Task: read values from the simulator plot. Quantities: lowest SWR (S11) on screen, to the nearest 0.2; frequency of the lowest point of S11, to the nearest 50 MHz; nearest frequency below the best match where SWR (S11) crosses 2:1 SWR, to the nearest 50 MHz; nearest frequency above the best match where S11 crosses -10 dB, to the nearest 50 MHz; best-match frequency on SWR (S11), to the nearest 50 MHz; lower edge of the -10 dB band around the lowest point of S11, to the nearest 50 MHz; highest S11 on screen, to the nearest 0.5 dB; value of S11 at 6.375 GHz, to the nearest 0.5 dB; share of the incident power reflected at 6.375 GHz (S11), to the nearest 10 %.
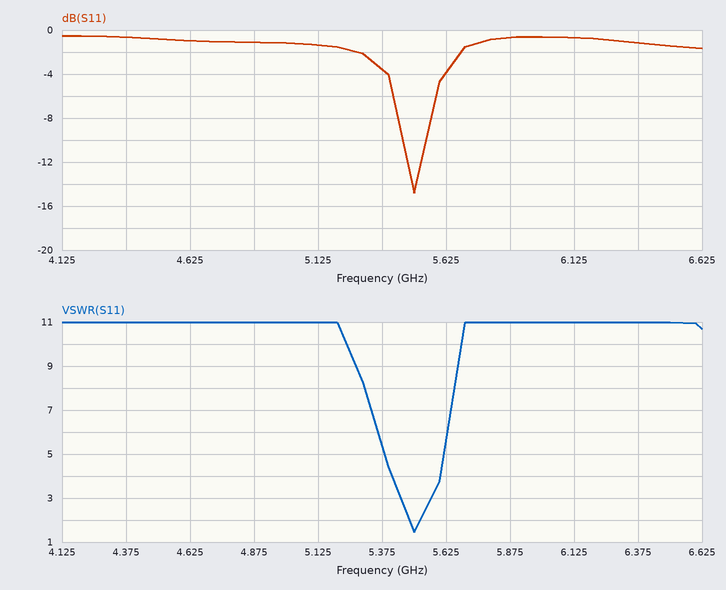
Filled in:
1.4
5.50 GHz
5.50 GHz
5.55 GHz
5.50 GHz
5.45 GHz
-0.5 dB
-1.0 dB
80 %
